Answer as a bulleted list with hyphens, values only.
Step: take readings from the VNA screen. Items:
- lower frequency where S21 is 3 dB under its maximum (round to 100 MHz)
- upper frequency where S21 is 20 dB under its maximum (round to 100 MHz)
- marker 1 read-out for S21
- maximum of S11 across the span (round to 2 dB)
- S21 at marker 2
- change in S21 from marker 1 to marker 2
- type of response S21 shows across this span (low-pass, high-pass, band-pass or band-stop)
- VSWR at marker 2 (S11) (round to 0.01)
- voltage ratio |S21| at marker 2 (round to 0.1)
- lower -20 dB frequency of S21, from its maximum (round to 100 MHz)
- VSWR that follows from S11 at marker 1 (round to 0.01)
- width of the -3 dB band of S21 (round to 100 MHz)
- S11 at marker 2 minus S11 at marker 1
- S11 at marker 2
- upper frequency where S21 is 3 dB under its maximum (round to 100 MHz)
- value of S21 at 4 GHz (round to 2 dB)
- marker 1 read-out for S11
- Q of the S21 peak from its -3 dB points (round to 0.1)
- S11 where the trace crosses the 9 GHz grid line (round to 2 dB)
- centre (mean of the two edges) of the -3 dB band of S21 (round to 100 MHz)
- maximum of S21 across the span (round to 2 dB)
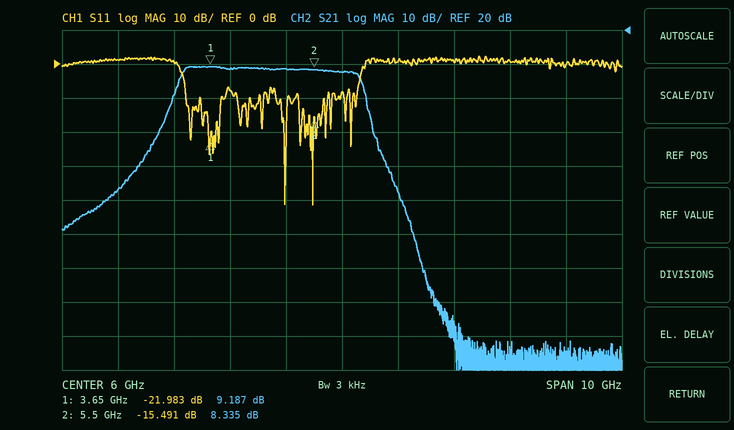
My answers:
- 3.1 GHz
- 6.6 GHz
- 9.187 dB
- 2 dB
- 8.335 dB
- -0.852 dB
- band-pass
- 1.40
- 2.6
- 2.7 GHz
- 1.17
- 3.2 GHz
- 6.492 dB
- -15.491 dB
- 6.3 GHz
- 8 dB
- -21.983 dB
- 1.5
- 0 dB
- 4.7 GHz
- 10 dB
